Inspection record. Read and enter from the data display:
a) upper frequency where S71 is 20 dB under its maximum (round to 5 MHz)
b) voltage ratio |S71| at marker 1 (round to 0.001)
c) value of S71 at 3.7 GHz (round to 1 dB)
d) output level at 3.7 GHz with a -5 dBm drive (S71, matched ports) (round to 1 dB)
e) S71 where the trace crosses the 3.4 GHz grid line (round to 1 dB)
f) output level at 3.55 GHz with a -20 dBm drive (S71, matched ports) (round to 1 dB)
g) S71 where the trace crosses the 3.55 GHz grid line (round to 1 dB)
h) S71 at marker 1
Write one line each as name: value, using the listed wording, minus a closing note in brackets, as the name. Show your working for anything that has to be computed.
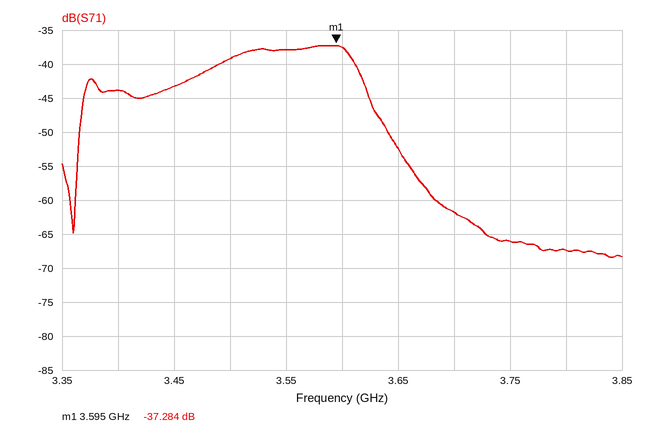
upper frequency where S71 is 20 dB under its maximum: 3.670 GHz
voltage ratio |S71| at marker 1: 10^(-37.284/20) ≈ 0.014
value of S71 at 3.7 GHz: -62 dB
output level at 3.7 GHz with a -5 dBm drive (S71, matched ports): -5 dBm + (-62 dB) = -67 dBm
S71 where the trace crosses the 3.4 GHz grid line: -44 dB
output level at 3.55 GHz with a -20 dBm drive (S71, matched ports): -20 dBm + (-38 dB) = -58 dBm
S71 where the trace crosses the 3.55 GHz grid line: -38 dB
S71 at marker 1: -37.284 dB
